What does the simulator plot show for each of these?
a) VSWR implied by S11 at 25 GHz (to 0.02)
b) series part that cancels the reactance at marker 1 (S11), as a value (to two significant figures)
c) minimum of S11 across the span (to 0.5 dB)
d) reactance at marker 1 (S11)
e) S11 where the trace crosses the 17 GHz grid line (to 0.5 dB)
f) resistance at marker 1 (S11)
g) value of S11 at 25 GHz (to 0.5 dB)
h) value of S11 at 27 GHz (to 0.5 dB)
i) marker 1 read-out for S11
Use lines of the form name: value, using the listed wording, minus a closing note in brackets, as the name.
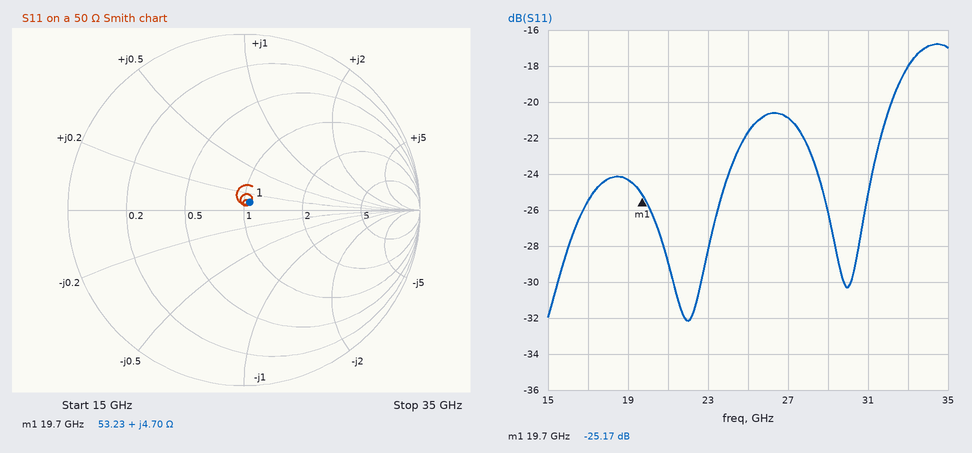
VSWR implied by S11 at 25 GHz: 1.18
series part that cancels the reactance at marker 1 (S11), as a value: 1.7 pF
minimum of S11 across the span: -32.0 dB
reactance at marker 1: +4.70 Ω
S11 where the trace crosses the 17 GHz grid line: -25.5 dB
resistance at marker 1: 53.23 Ω
value of S11 at 25 GHz: -21.5 dB
value of S11 at 27 GHz: -21.0 dB
marker 1 read-out for S11: -25.17 dB
